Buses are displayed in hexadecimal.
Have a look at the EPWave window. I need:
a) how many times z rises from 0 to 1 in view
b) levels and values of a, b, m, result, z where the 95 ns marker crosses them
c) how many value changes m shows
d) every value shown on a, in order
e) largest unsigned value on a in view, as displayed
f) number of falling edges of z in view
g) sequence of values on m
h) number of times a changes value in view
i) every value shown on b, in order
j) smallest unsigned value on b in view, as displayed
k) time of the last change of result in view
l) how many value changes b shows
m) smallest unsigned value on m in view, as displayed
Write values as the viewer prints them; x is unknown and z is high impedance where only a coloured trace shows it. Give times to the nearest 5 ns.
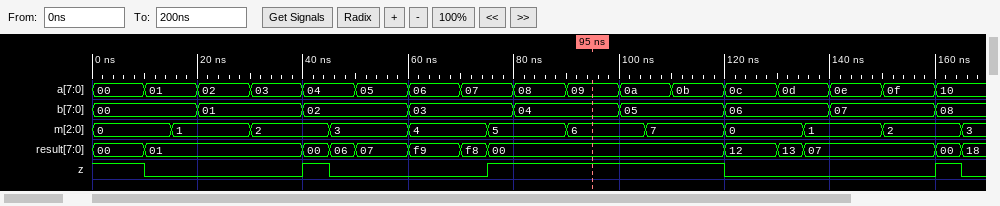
3
a=09, b=04, m=6, result=00, z=1
11
00, 01, 02, 03, 04, 05, 06, 07, 08, 09, 0a, 0b, 0c, 0d, 0e, 0f, 10
10
4
0, 1, 2, 3, 4, 5, 6, 7, 0, 1, 2, 3
16
00, 01, 02, 03, 04, 05, 06, 07, 08
00
165 ns
8
0
